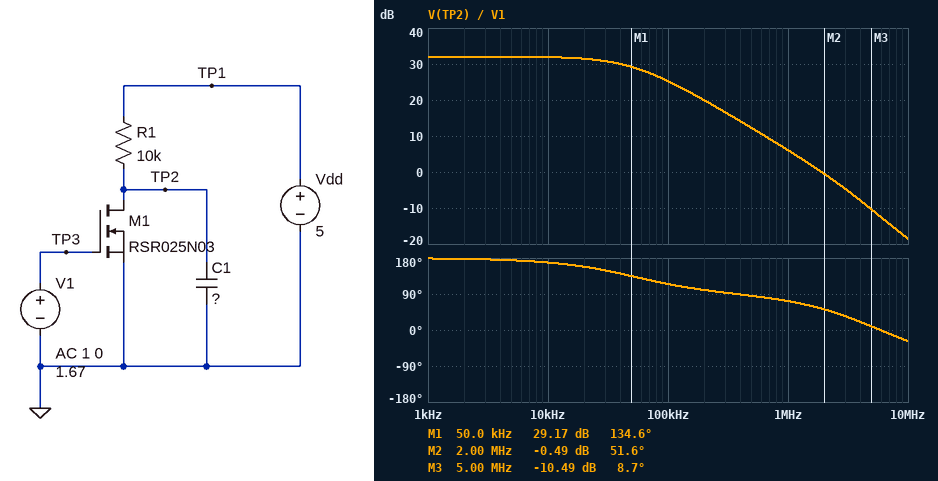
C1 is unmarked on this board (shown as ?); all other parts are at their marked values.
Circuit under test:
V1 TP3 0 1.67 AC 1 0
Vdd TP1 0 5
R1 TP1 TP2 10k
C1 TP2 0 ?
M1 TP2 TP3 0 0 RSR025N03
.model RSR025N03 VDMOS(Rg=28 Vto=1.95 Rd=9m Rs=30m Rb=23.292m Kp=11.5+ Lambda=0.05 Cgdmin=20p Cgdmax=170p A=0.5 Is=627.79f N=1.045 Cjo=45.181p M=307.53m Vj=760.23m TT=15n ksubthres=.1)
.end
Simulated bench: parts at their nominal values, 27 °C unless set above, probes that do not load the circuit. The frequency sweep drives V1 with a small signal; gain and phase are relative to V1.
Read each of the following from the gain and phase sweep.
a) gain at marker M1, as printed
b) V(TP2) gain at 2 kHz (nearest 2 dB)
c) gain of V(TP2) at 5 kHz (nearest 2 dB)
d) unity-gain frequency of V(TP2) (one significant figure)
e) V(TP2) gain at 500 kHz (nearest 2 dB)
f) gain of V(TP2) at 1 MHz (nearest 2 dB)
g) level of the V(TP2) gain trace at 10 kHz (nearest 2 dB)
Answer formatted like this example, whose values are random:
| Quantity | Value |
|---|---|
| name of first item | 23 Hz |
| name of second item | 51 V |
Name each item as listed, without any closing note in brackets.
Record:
| Quantity | Value |
|---|---|
| gain at marker M1, as printed | 29.17 dB |
| V(TP2) gain at 2 kHz | 32 dB |
| gain of V(TP2) at 5 kHz | 32 dB |
| unity-gain frequency of V(TP2) | 2 MHz |
| V(TP2) gain at 500 kHz | 12 dB |
| gain of V(TP2) at 1 MHz | 6 dB |
| level of the V(TP2) gain trace at 10 kHz | 32 dB |
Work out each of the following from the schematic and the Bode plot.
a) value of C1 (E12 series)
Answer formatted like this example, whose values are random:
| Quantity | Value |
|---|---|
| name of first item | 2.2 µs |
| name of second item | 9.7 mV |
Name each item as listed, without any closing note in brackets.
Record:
| Quantity | Value |
|---|---|
| value of C1 | 220 pF |
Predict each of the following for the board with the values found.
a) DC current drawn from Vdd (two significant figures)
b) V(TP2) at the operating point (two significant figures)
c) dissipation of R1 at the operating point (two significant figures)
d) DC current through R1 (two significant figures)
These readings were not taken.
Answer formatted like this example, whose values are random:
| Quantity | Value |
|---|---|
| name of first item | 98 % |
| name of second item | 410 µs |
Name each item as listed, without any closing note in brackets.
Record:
| Quantity | Value |
|---|---|
| DC current drawn from Vdd | 230 µA |
| V(TP2) at the operating point | 2.7 V |
| dissipation of R1 at the operating point | 520 µW |
| DC current through R1 | 230 µA |
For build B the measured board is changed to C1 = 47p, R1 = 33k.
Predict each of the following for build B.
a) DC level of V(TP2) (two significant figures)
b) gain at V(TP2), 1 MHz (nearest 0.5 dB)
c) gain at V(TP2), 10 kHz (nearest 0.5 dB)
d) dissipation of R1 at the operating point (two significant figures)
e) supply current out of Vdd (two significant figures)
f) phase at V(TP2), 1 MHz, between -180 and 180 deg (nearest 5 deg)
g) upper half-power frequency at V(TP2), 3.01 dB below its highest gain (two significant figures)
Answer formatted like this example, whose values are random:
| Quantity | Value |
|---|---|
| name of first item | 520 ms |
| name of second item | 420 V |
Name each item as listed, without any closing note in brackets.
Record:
| Quantity | Value |
|---|---|
| DC level of V(TP2) | 3.0 mV |
| gain at V(TP2), 1 MHz | -24.0 dB |
| gain at V(TP2), 10 kHz | -24.5 dB |
| dissipation of R1 at the operating point | 760 µW |
| supply current out of Vdd | 150 µA |
| phase at V(TP2), 1 MHz, between -180 and 180 deg | 135 deg |
| upper half-power frequency at V(TP2), 3.01 dB below its highest gain | 29 MHz |
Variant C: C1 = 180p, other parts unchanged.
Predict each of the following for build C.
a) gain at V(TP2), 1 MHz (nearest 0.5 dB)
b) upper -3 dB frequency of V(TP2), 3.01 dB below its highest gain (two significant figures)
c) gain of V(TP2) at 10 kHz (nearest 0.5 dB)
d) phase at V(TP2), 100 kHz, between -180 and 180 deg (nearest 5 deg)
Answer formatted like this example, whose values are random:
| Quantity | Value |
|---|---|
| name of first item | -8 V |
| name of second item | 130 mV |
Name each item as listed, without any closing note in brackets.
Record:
| Quantity | Value |
|---|---|
| gain at V(TP2), 1 MHz | 7.0 dB |
| upper -3 dB frequency of V(TP2), 3.01 dB below its highest gain | 58 kHz |
| gain of V(TP2) at 10 kHz | 32.0 dB |
| phase at V(TP2), 100 kHz, between -180 and 180 deg | 120 deg |
